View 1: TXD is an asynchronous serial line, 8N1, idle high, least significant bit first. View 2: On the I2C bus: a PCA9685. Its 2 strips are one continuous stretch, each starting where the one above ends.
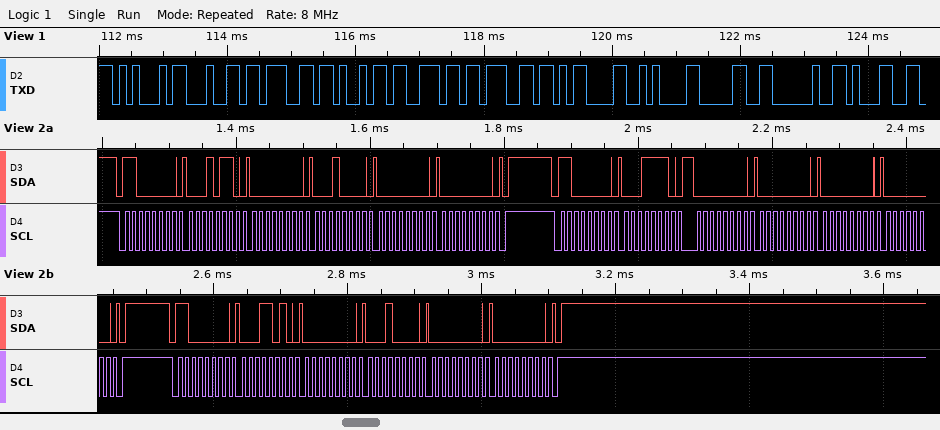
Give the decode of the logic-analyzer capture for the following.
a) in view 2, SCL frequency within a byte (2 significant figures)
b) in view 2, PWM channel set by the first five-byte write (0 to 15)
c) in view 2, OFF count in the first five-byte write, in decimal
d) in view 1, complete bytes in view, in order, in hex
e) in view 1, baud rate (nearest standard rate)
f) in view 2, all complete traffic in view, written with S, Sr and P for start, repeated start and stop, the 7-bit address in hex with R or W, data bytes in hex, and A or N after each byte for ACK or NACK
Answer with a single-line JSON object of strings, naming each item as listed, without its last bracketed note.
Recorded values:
{"in view 2, SCL frequency within a byte": "100 kHz", "in view 2, PWM channel set by the first five-byte write": "4", "in view 2, OFF count in the first five-byte write, in decimal": "0", "in view 1, complete bytes in view, in order, in hex": "45 64 67 69 6E 67 0D 0A 30 20 31", "in view 1, baud rate": "9600 baud", "in view 2, all complete traffic in view, written with S, Sr and P for start, repeated start and stop, the 7-bit address in hex with R or W, data bytes in hex, and A or N after each byte for ACK or NACK": "S 60W A 16 A 00 A 10 A 00 A 00 A P S 60W A 1E A 00 A 00 A 00 A 00 A P S 60W A 1A A 00 A 10 A 00 A 00 A P"}
